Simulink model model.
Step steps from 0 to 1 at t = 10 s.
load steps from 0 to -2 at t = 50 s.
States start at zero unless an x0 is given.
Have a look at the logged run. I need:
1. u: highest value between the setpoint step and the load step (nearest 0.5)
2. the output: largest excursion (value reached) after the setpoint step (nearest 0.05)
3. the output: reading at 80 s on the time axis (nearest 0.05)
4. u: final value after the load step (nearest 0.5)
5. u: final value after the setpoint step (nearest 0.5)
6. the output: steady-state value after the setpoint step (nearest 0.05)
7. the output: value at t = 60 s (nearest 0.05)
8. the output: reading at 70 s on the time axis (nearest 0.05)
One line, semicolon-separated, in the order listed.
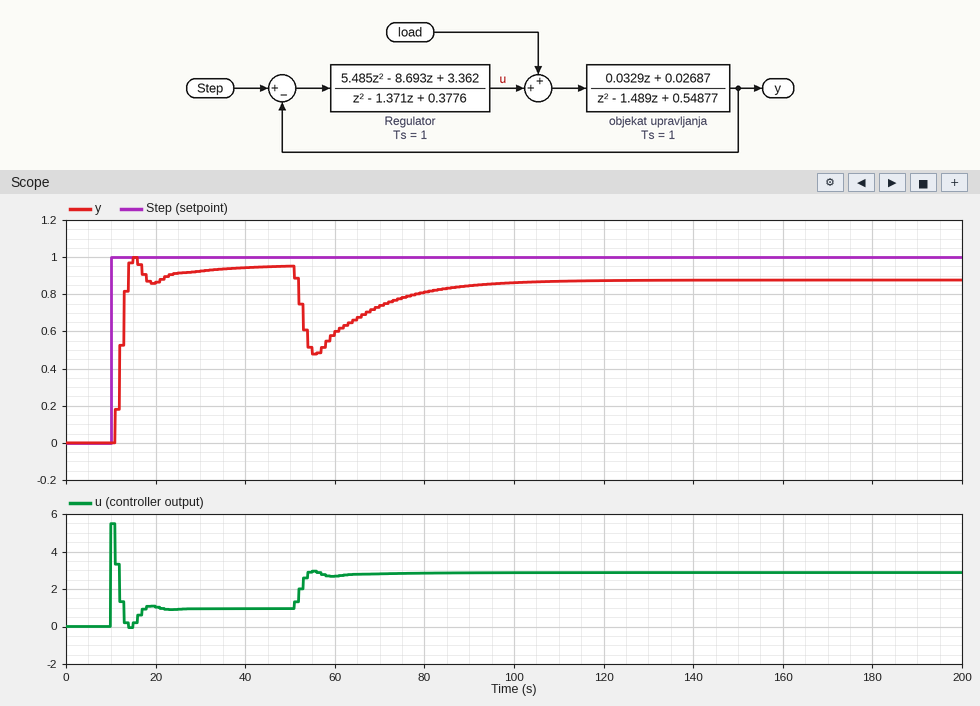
5.5; 1.00; 0.80; 3.0; 1.0; 0.95; 0.60; 0.75
